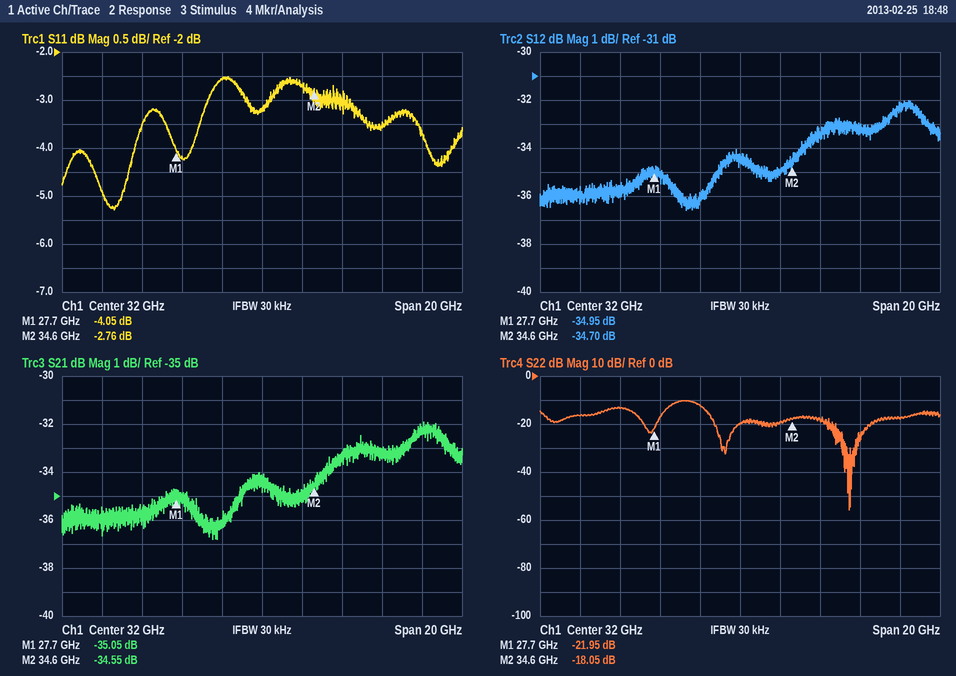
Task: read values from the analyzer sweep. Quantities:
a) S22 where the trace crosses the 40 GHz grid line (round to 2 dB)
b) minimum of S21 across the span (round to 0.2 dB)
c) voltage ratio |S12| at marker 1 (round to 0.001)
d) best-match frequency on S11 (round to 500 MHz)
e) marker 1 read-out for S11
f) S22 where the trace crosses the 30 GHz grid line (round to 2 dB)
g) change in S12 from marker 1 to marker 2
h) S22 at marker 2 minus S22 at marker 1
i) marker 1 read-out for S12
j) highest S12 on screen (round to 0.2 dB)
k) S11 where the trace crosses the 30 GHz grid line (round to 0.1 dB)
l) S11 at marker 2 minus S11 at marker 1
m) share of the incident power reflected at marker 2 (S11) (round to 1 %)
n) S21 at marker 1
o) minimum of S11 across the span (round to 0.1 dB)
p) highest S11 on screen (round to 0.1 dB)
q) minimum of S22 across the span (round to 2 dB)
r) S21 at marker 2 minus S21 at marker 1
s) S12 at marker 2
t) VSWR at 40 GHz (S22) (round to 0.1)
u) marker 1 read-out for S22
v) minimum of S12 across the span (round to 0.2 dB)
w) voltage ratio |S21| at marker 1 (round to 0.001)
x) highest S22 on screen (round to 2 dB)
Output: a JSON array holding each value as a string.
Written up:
["-18 dB", "-36.8 dB", "0.018", "24.5 GHz", "-4.05 dB", "-12 dB", "0.25 dB", "3.90 dB", "-34.95 dB", "-32.0 dB", "-2.6 dB", "1.29 dB", "53 %", "-35.05 dB", "-5.3 dB", "-2.5 dB", "-56 dB", "0.50 dB", "-34.70 dB", "1.3", "-21.95 dB", "-36.6 dB", "0.018", "-10 dB"]
